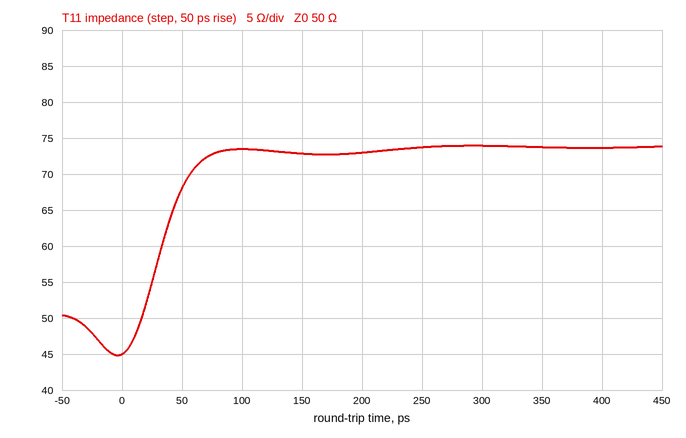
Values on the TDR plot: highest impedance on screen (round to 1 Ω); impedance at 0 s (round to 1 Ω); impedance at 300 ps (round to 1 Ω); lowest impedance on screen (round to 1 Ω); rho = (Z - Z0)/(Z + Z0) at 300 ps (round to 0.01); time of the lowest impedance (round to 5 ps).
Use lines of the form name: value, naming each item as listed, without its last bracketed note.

highest impedance on screen: 74 Ω
impedance at 0 s: 45 Ω
impedance at 300 ps: 74 Ω
lowest impedance on screen: 45 Ω
rho = (Z - Z0)/(Z + Z0) at 300 ps: +0.19
time of the lowest impedance: -5 ps
